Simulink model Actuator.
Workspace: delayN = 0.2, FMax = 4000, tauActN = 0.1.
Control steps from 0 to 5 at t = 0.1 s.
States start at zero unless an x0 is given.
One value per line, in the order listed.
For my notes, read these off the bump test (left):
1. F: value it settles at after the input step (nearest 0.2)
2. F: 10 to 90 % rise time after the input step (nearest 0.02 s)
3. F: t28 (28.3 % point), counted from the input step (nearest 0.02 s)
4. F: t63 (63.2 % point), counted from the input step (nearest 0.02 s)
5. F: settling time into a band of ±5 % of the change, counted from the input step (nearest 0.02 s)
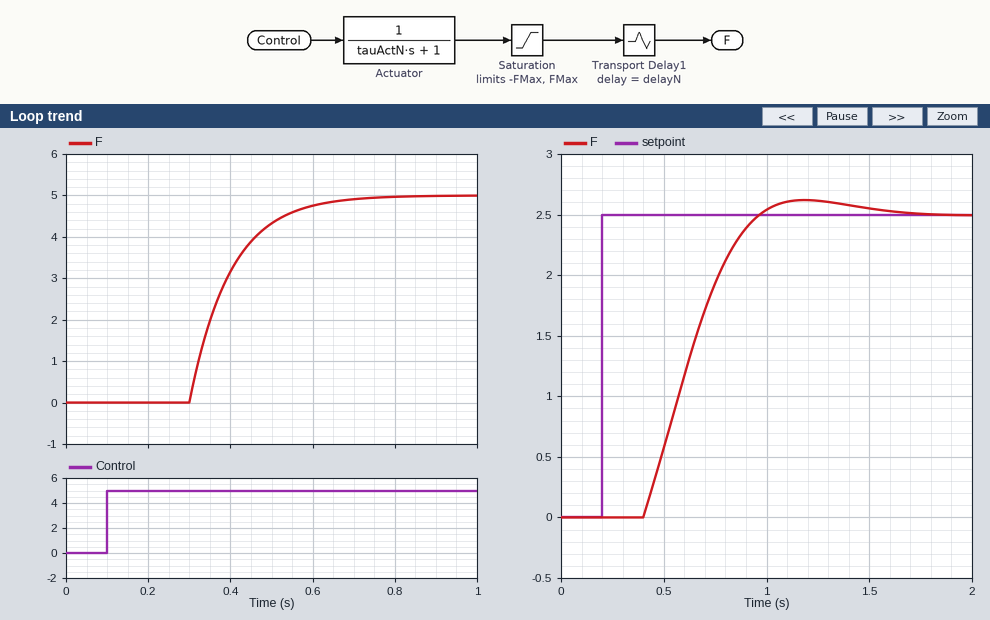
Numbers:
5.0
0.22 s
0.24 s
0.30 s
0.50 s
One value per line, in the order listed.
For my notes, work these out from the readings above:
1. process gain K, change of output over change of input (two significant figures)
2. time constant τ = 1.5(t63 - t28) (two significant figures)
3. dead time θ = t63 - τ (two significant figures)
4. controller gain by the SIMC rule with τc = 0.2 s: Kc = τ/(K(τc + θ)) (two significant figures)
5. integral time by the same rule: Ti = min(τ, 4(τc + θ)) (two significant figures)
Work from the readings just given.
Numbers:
1.0
0.090 s
0.21 s
0.22
0.090 s
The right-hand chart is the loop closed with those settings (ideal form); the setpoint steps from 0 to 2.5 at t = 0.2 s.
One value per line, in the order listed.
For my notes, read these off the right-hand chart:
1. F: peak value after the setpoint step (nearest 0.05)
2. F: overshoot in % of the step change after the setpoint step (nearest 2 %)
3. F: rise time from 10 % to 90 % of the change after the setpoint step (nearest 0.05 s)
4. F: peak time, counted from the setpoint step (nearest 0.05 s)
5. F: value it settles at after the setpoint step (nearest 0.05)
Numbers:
2.60
4 %
0.40 s
1.00 s
2.50
